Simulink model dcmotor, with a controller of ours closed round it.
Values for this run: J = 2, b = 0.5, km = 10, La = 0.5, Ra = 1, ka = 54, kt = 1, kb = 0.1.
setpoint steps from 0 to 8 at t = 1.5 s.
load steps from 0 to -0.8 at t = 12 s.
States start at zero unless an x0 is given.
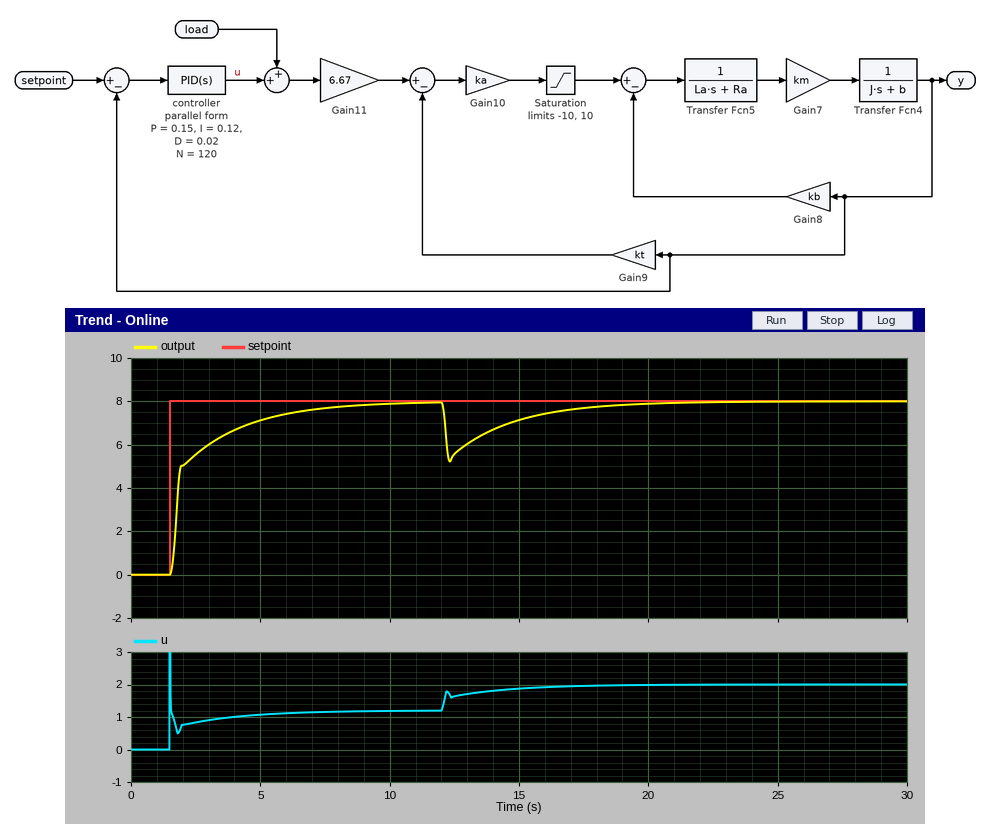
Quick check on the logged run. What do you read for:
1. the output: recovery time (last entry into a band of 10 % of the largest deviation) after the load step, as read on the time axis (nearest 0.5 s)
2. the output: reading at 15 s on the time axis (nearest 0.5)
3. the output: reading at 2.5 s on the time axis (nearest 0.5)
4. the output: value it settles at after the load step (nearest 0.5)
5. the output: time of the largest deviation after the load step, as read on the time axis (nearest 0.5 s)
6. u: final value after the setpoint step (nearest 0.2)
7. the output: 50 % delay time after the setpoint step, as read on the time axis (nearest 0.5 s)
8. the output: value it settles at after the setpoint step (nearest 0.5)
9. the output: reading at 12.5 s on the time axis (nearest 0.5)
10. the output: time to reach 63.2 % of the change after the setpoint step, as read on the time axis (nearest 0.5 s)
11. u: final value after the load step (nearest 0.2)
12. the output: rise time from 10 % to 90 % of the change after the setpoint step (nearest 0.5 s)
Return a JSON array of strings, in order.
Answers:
["18.0 s", "7.0", "5.5", "8.0", "12.5 s", "1.2", "2.0 s", "8.0", "5.5", "2.0 s", "2.0", "3.5 s"]
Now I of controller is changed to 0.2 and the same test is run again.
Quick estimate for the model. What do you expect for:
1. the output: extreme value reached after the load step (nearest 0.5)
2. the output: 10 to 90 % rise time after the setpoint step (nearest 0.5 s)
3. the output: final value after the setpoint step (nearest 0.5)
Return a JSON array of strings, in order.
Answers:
["5.5", "2.0 s", "8.0"]
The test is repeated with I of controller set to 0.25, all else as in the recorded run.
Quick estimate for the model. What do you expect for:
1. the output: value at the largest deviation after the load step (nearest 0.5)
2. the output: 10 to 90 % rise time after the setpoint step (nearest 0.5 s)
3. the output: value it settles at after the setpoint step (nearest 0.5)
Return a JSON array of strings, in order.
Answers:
["5.5", "1.5 s", "8.0"]
